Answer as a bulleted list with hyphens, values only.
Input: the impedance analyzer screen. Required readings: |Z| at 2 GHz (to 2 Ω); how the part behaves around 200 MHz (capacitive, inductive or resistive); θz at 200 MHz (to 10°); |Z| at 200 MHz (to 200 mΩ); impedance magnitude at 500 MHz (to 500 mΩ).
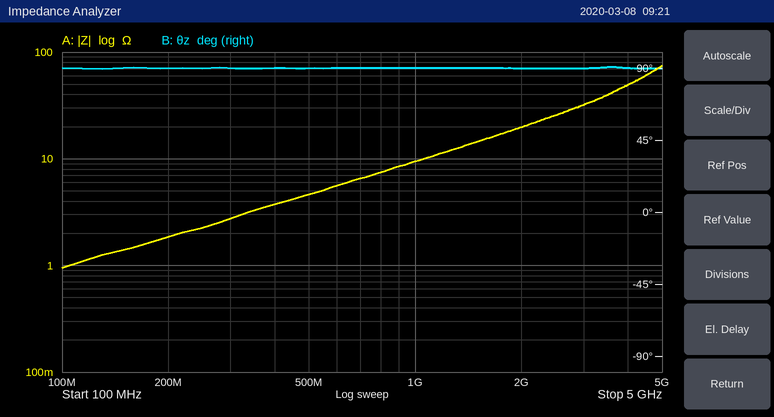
- 20 Ω
- inductive
- 90°
- 1.8 Ω
- 4.5 Ω
